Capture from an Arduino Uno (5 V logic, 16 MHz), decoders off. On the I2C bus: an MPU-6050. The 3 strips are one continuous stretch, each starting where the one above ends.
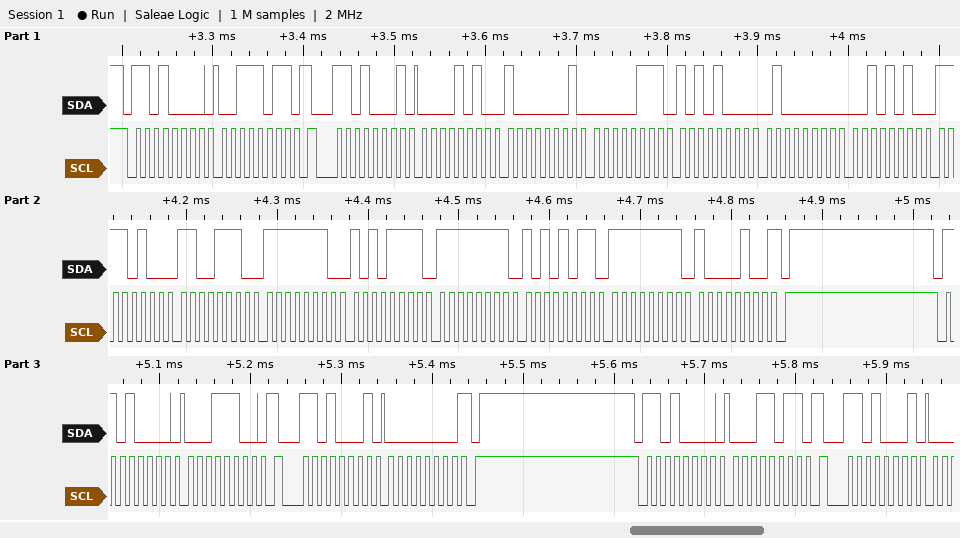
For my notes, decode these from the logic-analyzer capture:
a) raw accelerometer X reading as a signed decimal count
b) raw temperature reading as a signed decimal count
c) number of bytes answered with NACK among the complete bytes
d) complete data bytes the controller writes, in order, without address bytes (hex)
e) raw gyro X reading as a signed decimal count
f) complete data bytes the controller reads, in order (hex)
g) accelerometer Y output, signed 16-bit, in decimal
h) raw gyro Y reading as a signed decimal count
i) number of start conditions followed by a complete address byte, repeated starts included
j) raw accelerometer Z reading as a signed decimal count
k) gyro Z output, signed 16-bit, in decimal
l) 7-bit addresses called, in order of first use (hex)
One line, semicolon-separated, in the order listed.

2689; -2866; 2; 3B 1C 1B; -337; 0A 81 07 A8 40 2A F4 CE FE AF FF AB FF 84 00; 1960; -85; 6; 16426; -124; 0x68
